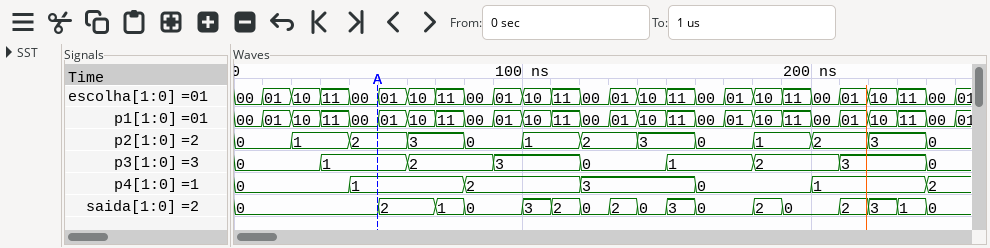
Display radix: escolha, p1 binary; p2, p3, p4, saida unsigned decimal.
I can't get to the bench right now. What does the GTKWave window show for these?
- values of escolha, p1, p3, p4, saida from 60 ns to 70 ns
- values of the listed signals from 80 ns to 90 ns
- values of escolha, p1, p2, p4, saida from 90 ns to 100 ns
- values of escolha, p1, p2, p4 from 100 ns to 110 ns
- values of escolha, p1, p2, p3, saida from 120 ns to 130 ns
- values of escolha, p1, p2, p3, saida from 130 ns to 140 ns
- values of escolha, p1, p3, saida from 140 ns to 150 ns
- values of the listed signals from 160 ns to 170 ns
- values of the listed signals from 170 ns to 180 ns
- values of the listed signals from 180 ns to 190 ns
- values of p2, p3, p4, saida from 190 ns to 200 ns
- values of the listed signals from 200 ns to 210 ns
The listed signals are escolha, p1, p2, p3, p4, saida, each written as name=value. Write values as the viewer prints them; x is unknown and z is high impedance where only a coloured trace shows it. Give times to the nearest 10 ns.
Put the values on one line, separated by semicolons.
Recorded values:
escolha=10, p1=10, p3=2, p4=1, saida=2; escolha=00, p1=00, p2=0, p3=2, p4=2, saida=0; escolha=01, p1=01, p2=0, p4=2, saida=0; escolha=10, p1=10, p2=1, p4=2; escolha=00, p1=00, p2=2, p3=0, saida=0; escolha=01, p1=01, p2=2, p3=0, saida=2; escolha=10, p1=10, p3=0, saida=0; escolha=00, p1=00, p2=0, p3=1, p4=0, saida=0; escolha=01, p1=01, p2=0, p3=1, p4=0, saida=0; escolha=10, p1=10, p2=1, p3=2, p4=0, saida=2; p2=1, p3=2, p4=0, saida=0; escolha=00, p1=00, p2=2, p3=2, p4=1, saida=0
